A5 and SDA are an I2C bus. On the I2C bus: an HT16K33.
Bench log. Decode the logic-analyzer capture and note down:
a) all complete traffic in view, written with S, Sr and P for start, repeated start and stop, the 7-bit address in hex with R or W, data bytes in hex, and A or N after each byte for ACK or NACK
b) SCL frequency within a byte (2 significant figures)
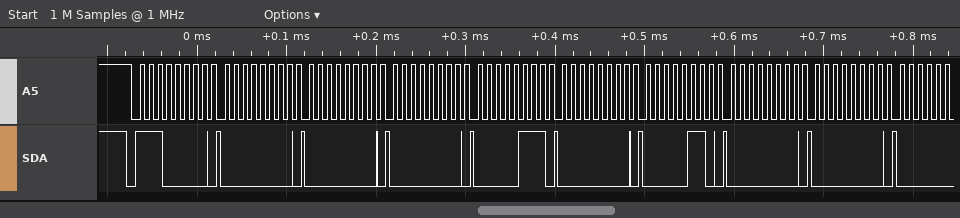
S 70W A 00 A 00 A 00 A 07 A 00 A 06 A 00 A 00 A
100 kHz
